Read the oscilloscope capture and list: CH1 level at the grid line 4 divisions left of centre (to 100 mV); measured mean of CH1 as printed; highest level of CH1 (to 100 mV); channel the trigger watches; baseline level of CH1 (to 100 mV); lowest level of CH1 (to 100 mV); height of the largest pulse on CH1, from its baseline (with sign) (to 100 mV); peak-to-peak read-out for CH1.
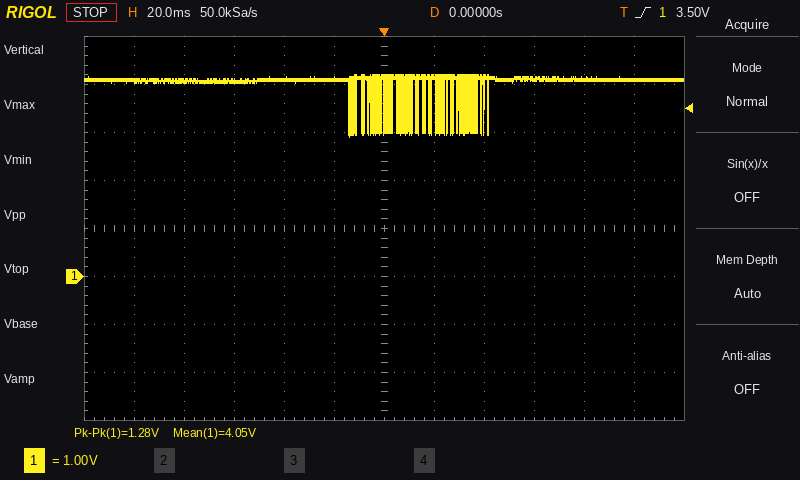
4.1 V
4.05 V
4.2 V
CH1
4.1 V
2.9 V
-1.2 V
1.28 V
